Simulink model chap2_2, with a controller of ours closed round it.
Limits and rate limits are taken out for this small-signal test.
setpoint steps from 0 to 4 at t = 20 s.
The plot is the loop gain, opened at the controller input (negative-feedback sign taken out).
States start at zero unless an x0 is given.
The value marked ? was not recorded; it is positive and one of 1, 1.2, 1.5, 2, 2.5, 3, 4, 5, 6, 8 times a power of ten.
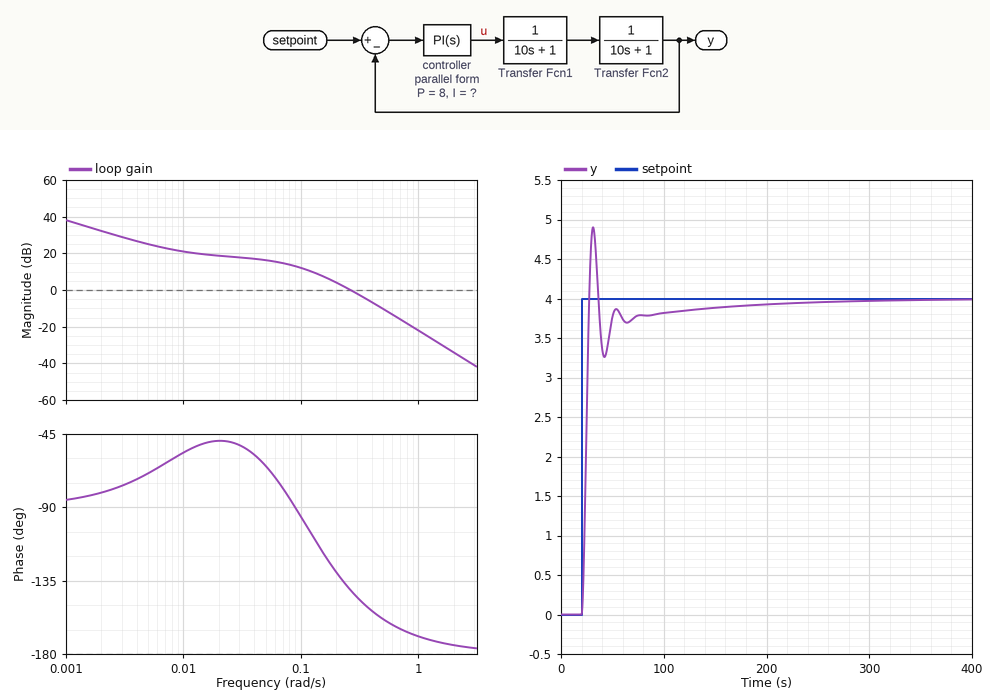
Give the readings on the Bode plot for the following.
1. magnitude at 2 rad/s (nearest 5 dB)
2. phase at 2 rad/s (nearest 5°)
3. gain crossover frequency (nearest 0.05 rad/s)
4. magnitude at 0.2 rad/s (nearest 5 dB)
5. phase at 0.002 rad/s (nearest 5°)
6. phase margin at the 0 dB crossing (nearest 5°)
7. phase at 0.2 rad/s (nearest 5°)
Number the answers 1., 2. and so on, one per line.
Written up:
1. -35 dB
2. -175°
3. 0.25 rad/s
4. 5 dB
5. -80°
6. 40°
7. -130°
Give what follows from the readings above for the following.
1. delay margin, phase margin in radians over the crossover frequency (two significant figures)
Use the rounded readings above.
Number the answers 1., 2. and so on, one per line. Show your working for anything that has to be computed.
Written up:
1. 40 × π / 180 / 0.25 = 2.8 s
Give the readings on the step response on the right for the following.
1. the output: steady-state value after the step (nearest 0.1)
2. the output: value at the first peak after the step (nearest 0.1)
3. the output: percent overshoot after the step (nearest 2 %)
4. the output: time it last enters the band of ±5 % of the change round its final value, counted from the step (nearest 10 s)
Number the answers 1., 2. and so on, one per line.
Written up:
1. 4.0
2. 4.9
3. 22 %
4. 70 s
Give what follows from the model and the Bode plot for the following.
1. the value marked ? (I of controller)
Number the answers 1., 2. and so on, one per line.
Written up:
1. 0.08
